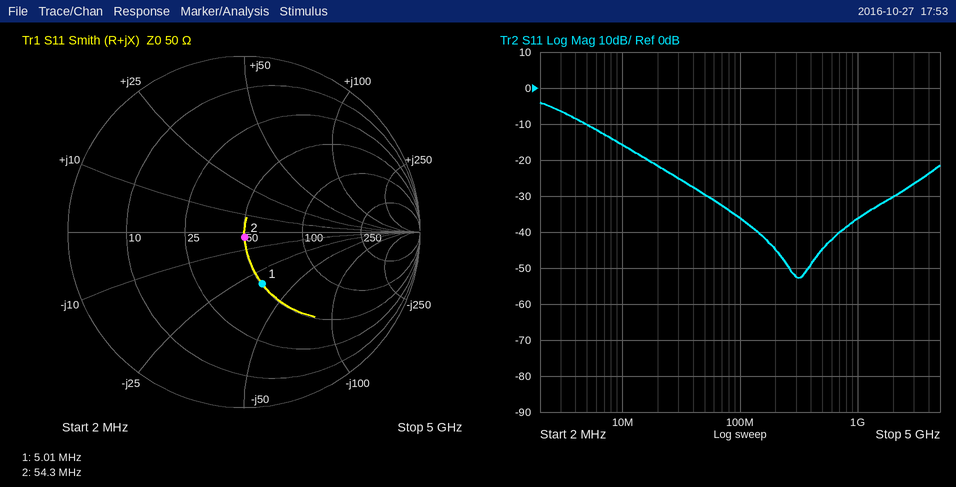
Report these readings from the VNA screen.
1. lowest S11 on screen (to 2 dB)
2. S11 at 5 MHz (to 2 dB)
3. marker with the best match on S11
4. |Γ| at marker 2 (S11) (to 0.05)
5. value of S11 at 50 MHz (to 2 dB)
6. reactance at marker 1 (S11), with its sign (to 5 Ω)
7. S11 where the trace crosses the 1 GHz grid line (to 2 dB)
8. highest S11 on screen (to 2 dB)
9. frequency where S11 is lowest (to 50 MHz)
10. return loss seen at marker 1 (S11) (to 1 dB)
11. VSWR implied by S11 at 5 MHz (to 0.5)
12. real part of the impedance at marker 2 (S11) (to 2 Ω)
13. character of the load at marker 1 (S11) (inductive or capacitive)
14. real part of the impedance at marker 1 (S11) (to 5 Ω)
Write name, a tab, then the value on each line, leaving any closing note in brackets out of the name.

lowest S11 on screen	-52 dB
S11 at 5 MHz	-10 dB
marker with the best match on S11	marker 2
|Γ| at marker 2 (S11)	0.05
value of S11 at 50 MHz	-30 dB
reactance at marker 1 (S11), with its sign	-35 Ω
S11 where the trace crosses the 1 GHz grid line	-36 dB
highest S11 on screen	-4 dB
frequency where S11 is lowest	300 MHz
return loss seen at marker 1 (S11)	10 dB
VSWR implied by S11 at 5 MHz	2.0
real part of the impedance at marker 2 (S11)	50 Ω
character of the load at marker 1 (S11)	capacitive
real part of the impedance at marker 1 (S11)	50 Ω
